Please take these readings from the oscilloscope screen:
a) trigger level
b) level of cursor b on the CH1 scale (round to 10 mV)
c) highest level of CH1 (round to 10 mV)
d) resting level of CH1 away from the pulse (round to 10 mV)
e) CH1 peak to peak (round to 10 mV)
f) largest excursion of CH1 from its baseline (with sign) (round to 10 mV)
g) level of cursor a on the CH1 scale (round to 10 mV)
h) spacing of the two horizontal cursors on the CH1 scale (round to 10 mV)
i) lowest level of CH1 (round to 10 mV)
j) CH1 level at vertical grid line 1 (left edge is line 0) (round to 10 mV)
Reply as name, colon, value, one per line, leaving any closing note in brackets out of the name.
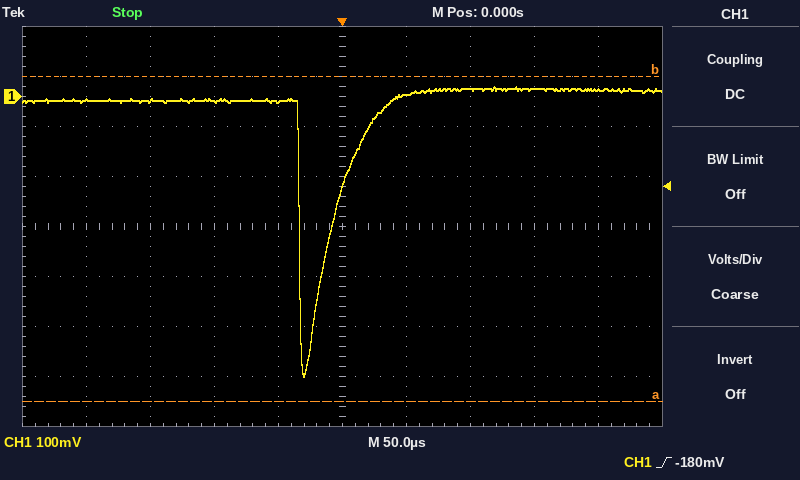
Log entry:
trigger level: -180 mV
level of cursor b on the CH1 scale: 40 mV
highest level of CH1: 20 mV
resting level of CH1 away from the pulse: -10 mV
CH1 peak to peak: 580 mV
largest excursion of CH1 from its baseline (with sign): -550 mV
level of cursor a on the CH1 scale: -610 mV
spacing of the two horizontal cursors on the CH1 scale: 650 mV
lowest level of CH1: -560 mV
CH1 level at vertical grid line 1 (left edge is line 0): -10 mV
